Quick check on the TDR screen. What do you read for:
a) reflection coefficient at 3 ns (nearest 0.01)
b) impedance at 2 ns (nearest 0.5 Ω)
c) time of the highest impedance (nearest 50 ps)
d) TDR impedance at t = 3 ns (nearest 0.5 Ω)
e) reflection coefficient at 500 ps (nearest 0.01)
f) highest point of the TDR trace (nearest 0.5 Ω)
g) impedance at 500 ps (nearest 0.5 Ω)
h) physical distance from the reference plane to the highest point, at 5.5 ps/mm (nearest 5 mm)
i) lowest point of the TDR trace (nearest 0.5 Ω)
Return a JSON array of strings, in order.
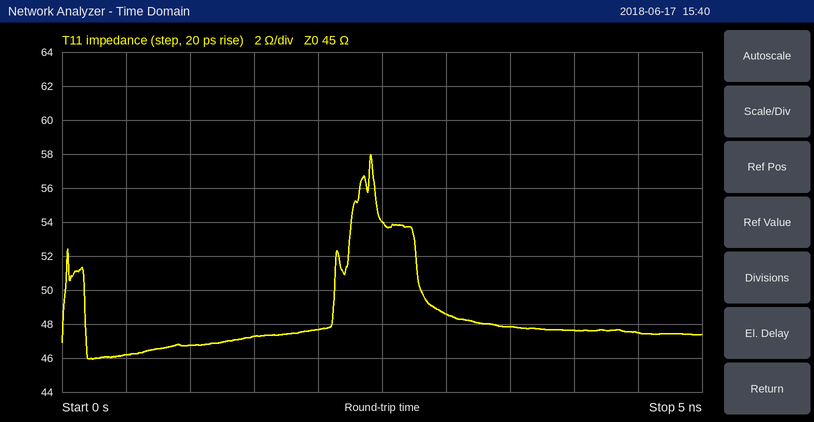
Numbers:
["+0.04", "47.5 Ω", "2.40 ns", "48.5 Ω", "+0.01", "58.0 Ω", "46.0 Ω", "220 mm", "46.0 Ω"]
